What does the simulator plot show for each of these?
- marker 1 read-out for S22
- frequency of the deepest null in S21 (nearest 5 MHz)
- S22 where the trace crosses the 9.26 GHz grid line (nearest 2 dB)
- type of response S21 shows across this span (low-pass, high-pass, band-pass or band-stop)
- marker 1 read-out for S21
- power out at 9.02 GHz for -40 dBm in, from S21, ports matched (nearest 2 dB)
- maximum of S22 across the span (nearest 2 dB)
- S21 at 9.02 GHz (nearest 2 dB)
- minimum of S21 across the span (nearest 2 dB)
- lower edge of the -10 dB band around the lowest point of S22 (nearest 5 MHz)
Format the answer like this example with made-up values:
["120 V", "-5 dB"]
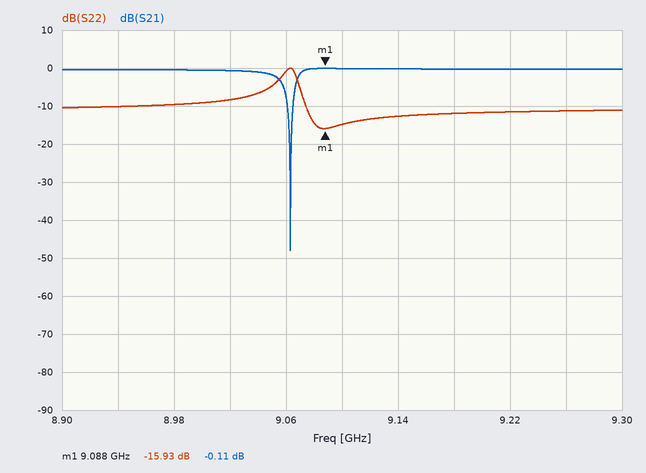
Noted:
["-15.93 dB", "9.065 GHz", "-12 dB", "band-stop", "-0.11 dB", "-40 dBm", "0 dB", "0 dB", "-48 dB", "9.075 GHz"]
